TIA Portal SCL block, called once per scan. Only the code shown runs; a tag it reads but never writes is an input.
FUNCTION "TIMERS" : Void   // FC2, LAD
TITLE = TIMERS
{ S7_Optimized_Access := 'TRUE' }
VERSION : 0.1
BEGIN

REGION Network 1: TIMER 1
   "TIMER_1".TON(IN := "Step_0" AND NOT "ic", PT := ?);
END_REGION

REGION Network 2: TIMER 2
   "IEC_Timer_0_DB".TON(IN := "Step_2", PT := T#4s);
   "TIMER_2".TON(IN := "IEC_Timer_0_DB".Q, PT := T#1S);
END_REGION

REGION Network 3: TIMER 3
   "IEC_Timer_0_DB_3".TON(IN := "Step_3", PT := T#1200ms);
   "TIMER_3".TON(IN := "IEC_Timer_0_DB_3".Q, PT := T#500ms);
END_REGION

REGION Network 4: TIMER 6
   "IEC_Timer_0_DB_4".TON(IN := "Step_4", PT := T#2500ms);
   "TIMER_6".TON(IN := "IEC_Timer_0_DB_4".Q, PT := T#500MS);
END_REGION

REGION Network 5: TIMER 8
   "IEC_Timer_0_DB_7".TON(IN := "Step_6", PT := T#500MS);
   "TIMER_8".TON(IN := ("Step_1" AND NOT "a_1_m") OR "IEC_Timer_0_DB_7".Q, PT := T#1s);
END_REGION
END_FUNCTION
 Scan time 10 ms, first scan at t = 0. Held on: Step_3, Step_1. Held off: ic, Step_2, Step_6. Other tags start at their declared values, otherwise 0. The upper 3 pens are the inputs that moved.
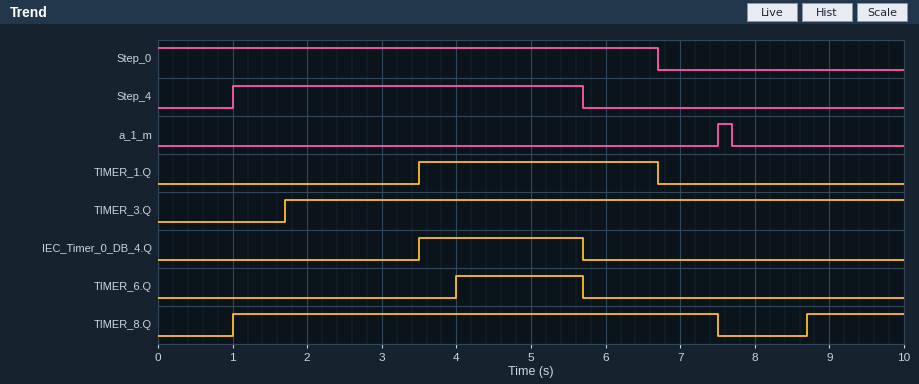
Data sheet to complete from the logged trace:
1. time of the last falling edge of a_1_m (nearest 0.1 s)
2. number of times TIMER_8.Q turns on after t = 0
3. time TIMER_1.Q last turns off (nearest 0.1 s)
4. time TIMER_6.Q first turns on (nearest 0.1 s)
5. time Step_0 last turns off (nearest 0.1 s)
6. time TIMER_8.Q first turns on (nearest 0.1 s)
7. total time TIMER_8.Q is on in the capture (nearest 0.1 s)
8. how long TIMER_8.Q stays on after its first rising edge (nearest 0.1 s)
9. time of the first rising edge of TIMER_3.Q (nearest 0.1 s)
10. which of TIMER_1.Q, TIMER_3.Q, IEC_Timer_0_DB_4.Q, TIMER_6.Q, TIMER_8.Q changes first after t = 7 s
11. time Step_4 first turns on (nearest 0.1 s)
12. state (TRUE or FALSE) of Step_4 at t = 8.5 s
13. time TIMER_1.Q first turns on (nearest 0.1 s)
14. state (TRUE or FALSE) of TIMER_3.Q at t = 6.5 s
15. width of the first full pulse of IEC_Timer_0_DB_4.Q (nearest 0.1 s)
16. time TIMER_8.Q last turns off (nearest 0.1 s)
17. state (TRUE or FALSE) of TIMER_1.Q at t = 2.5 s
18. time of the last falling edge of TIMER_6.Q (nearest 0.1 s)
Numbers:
7.7 s
2
6.7 s
4.0 s
6.7 s
1.0 s
7.8 s
6.5 s
1.7 s
TIMER_8.Q
1.0 s
FALSE
3.5 s
TRUE
2.2 s
7.5 s
FALSE
5.7 s
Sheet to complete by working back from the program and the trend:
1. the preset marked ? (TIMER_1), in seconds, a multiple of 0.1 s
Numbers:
3.5 s
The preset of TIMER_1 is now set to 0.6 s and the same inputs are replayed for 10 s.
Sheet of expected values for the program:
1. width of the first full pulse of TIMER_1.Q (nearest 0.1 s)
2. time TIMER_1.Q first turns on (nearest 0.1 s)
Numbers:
6.1 s
0.6 s
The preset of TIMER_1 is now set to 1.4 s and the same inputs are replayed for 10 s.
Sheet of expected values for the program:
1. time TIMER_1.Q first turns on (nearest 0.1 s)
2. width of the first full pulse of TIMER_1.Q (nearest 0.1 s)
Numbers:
1.4 s
5.3 s
